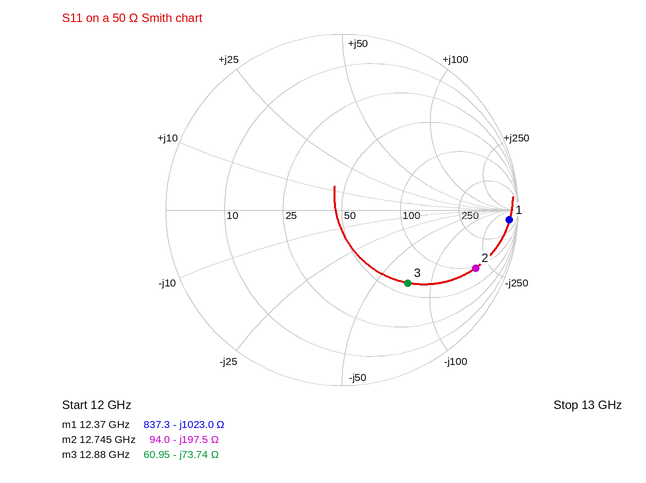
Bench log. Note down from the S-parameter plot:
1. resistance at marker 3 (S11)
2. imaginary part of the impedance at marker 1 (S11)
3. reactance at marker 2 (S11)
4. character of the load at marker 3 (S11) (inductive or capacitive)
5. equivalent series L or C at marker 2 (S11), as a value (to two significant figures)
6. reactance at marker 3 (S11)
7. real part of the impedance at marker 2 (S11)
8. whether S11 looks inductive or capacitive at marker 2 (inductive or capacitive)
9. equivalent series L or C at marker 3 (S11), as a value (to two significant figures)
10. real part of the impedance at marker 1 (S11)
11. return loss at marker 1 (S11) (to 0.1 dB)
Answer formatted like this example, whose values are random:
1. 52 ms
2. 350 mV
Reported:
1. 60.95 Ω
2. -1023.0 Ω
3. -197.5 Ω
4. capacitive
5. 63 fF
6. -73.74 Ω
7. 94.0 Ω
8. capacitive
9. 170 fF
10. 837.3 Ω
11. 0.4 dB
